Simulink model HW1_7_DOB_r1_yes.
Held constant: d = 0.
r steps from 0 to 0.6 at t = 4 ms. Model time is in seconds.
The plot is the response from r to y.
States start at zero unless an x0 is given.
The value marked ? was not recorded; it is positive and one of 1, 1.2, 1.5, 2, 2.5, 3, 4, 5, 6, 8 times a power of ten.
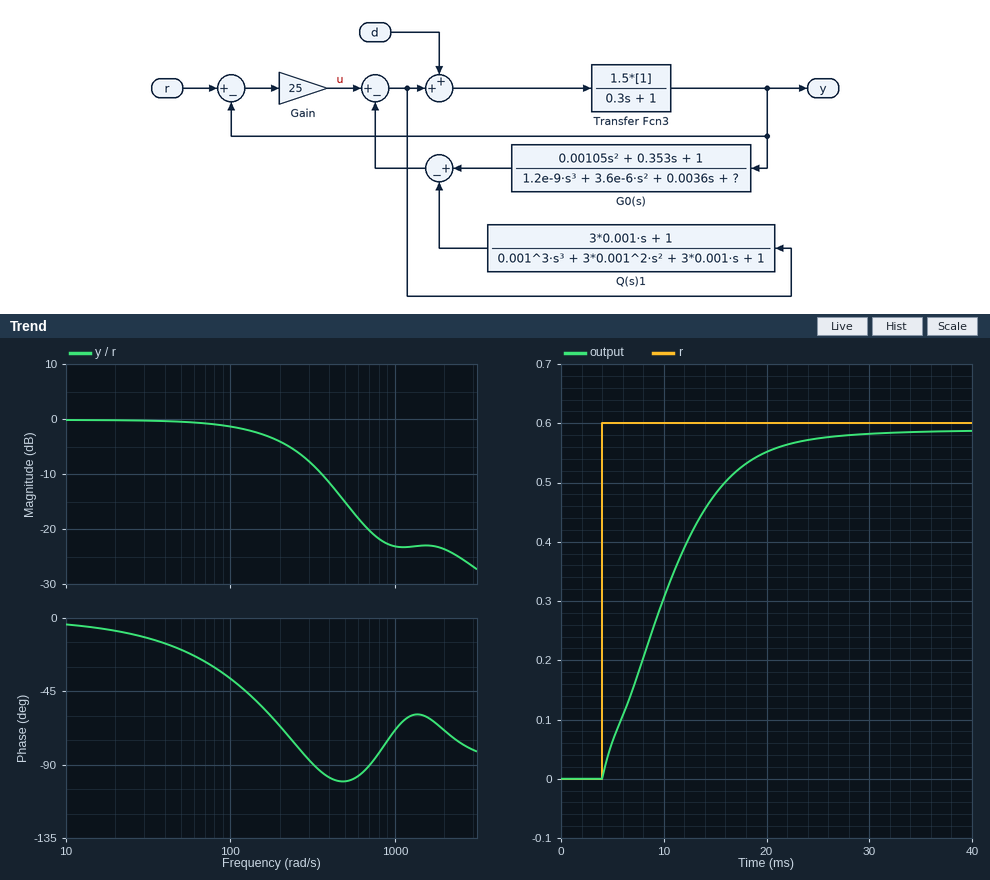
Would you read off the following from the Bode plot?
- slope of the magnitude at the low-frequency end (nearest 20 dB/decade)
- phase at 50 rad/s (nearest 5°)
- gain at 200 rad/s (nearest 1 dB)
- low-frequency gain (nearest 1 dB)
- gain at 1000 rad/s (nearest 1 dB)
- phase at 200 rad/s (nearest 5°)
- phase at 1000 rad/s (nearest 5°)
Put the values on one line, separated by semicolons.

0 dB/decade; -20°; -4 dB; 0 dB; -23 dB; -65°; -70°
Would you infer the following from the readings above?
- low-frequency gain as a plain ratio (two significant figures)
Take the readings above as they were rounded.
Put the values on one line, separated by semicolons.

1.0
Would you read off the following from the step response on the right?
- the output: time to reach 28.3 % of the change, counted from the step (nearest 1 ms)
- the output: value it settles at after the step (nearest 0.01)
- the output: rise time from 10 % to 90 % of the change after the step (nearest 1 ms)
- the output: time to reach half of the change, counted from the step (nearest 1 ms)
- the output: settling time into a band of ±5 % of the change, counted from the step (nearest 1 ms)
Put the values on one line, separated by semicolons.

3 ms; 0.59; 13 ms; 6 ms; 17 ms
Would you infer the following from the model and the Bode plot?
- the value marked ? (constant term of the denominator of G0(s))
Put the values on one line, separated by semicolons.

2
